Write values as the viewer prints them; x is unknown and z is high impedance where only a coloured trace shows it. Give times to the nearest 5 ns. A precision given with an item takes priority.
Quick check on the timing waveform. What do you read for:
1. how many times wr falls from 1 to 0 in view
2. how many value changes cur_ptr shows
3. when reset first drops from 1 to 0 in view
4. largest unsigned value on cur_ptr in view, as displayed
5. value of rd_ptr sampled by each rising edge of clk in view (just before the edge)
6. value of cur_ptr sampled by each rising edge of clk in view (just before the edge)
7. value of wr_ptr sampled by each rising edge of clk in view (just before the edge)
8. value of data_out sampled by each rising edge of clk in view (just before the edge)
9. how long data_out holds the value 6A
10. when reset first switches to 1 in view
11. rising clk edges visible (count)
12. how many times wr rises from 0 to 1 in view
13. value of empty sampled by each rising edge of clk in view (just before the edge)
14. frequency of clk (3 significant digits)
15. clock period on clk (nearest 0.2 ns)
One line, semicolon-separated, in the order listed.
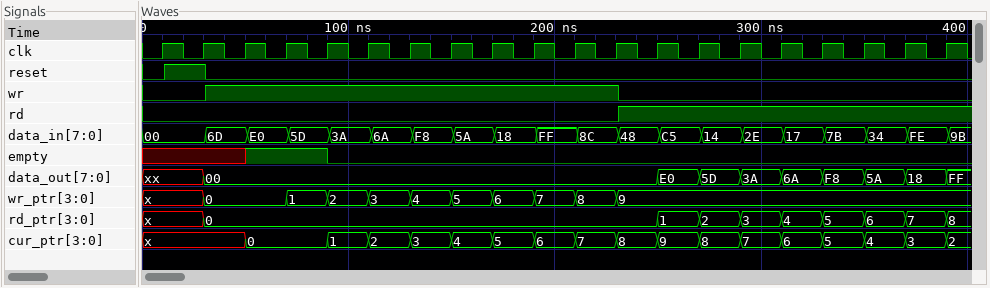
1; 17; 30 ns; 9; x, x, 0, 0, 0, 0, 0, 0, 0, 0, 0, 0, 0, 1, 2, 3, 4, 5, 6, 7; x, x, x, 0, 0, 1, 2, 3, 4, 5, 6, 7, 8, 9, 8, 7, 6, 5, 4, 3; x, x, 0, 0, 1, 2, 3, 4, 5, 6, 7, 8, 9, 9, 9, 9, 9, 9, 9, 9; xx, xx, 00, 00, 00, 00, 00, 00, 00, 00, 00, 00, 00, E0, 5D, 3A, 6A, F8, 5A, 18; 20 ns; 10 ns; 20; 1; x x x 1 1 0 0 0 0 0 0 0 0 0 0 0 0 0 0 0; 50.0 MHz; 20 ns
